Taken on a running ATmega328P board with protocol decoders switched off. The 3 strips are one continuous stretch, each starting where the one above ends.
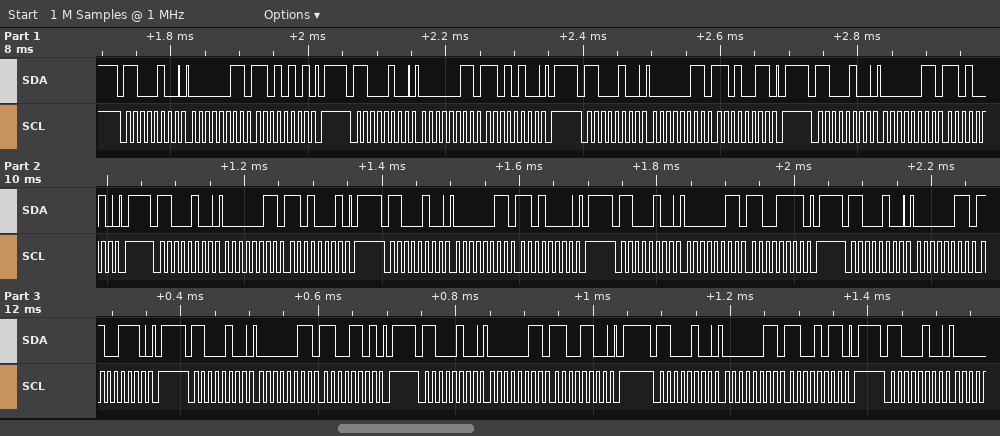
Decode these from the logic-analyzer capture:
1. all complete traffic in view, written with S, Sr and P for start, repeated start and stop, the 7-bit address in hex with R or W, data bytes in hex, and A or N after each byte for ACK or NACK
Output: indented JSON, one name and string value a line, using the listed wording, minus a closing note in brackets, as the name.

{
  "all complete traffic in view, written with S, Sr and P for start, repeated start and stop, the 7-bit address in hex with R or W, data bytes in hex, and A or N after each byte for ACK or NACK": "S 62W A 03 A D5 A P S 62W A 03 A D4 A P S 62W A 03 A D3 A P S 62W A 03 A D2 A P S 62W A 03 A D1 A P S 62W A 03 A D0 A P S 62W A 03 A CF A P S 62W A 03 A CE A P S 62W A 03 A CD A P S 62W A 03 A CC A P S 62W A 03 A CB A P S 62W A"
}
